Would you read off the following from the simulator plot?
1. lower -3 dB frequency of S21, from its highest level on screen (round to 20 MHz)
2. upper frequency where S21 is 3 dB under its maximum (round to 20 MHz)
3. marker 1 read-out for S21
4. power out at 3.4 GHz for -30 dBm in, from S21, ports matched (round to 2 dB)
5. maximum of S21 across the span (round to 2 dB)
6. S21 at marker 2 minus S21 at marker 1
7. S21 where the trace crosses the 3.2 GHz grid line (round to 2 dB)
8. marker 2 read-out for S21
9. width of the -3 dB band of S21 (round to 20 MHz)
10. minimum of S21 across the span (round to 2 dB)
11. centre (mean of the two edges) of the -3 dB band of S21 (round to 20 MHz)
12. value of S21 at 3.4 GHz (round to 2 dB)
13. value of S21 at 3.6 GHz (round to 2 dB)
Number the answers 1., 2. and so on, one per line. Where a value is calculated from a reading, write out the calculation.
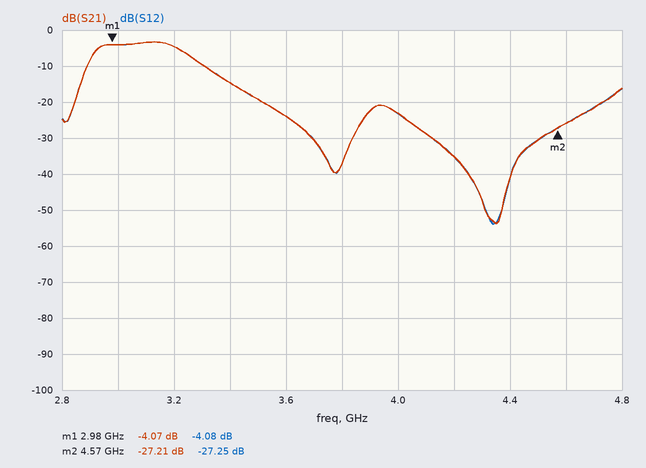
1. 2.92 GHz
2. 3.24 GHz
3. -4.07 dB
4. -30 dBm + (-14 dB) = -44 dBm
5. -4 dB
6. -27.21 − (-4.07) = -23.14 dB
7. -4 dB
8. -27.21 dB
9. 3.24 GHz − 2.92 GHz = 320 MHz
10. -54 dB
11. 3.08 GHz
12. -14 dB
13. -24 dB
